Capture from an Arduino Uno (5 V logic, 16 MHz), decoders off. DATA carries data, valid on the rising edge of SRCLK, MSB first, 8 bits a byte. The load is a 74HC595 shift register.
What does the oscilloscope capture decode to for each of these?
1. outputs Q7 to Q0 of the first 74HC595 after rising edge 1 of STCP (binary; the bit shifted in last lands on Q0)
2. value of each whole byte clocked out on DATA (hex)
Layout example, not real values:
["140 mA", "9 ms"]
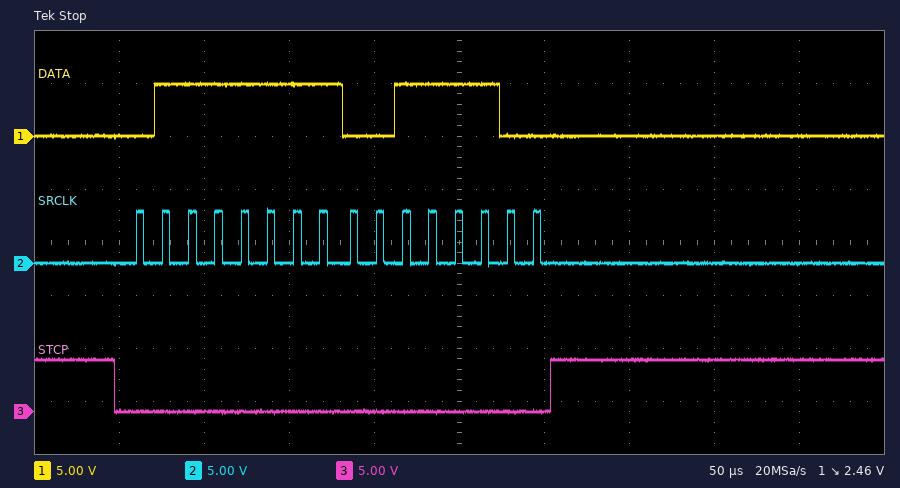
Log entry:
["00111100", "7F 3C"]
